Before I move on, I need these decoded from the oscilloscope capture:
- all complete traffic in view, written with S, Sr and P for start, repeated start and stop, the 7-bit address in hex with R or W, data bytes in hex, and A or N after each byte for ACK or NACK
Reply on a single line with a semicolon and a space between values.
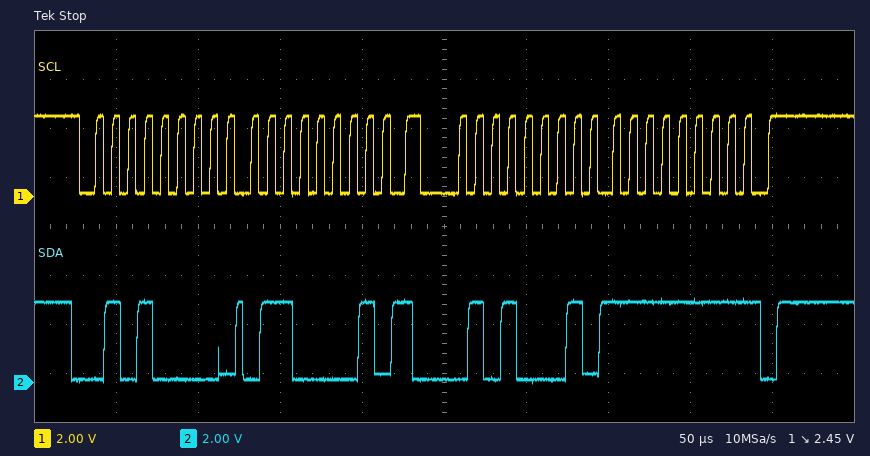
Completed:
S 28W A 61 A Sr 28R A FF N P
